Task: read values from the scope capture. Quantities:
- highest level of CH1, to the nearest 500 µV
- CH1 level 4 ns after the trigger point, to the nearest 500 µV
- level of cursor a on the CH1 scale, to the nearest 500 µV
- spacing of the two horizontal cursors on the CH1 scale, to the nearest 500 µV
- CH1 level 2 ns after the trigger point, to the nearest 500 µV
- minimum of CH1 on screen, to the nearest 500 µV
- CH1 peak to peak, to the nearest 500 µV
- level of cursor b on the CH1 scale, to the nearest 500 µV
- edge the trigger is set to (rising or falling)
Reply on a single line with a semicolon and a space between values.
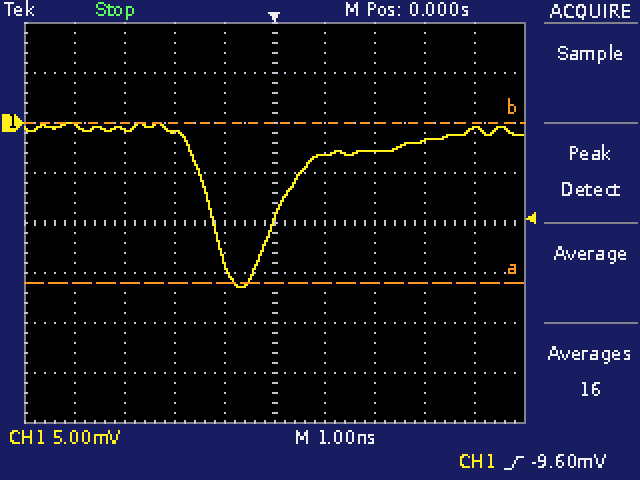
0.0 mV; -500 µV; -16.0 mV; 16.0 mV; -3.0 mV; -16.5 mV; 16.5 mV; 0.0 mV; rising
